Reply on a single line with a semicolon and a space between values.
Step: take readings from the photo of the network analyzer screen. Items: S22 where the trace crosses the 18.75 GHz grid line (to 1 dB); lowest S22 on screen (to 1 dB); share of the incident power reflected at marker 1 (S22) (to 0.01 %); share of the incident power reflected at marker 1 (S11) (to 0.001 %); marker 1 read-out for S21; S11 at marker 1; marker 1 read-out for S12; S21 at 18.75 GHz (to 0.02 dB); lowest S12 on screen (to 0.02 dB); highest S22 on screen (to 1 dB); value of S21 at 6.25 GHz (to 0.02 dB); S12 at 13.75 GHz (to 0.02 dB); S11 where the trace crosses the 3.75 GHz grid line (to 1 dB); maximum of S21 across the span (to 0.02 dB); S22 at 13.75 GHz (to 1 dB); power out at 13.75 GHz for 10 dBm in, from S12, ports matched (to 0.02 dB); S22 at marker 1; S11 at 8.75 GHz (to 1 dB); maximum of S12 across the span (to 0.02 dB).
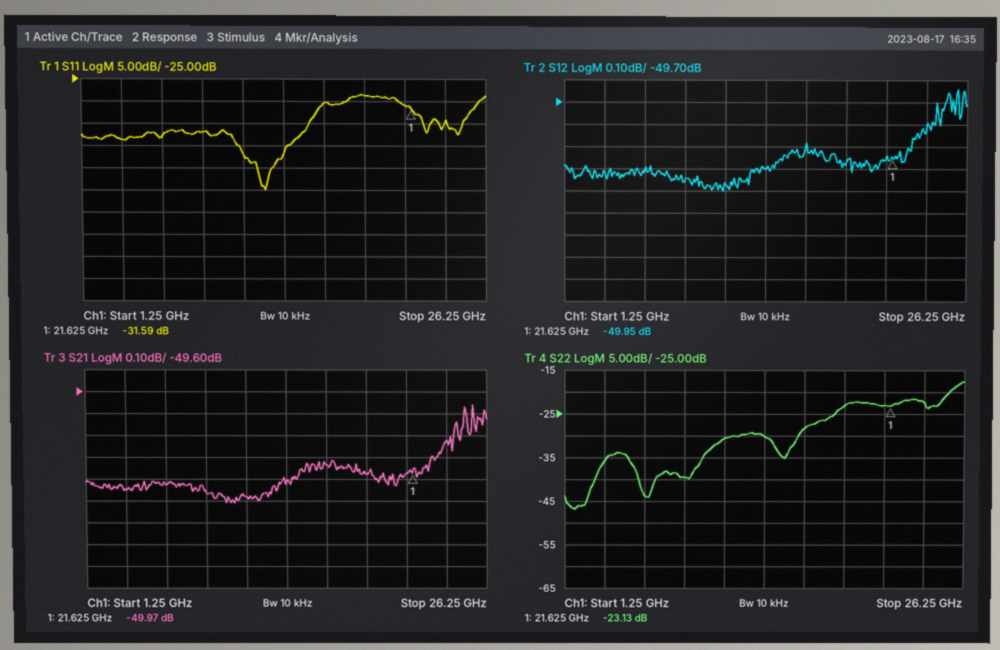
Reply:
-23 dB; -47 dB; 0.49 %; 0.069 %; -49.97 dB; -31.59 dB; -49.95 dB; -49.98 dB; -50.10 dB; -18 dB; -50.02 dB; -50.00 dB; -39 dB; -49.66 dB; -30 dB; -40.00 dBm; -23.13 dB; -37 dB; -49.64 dB
